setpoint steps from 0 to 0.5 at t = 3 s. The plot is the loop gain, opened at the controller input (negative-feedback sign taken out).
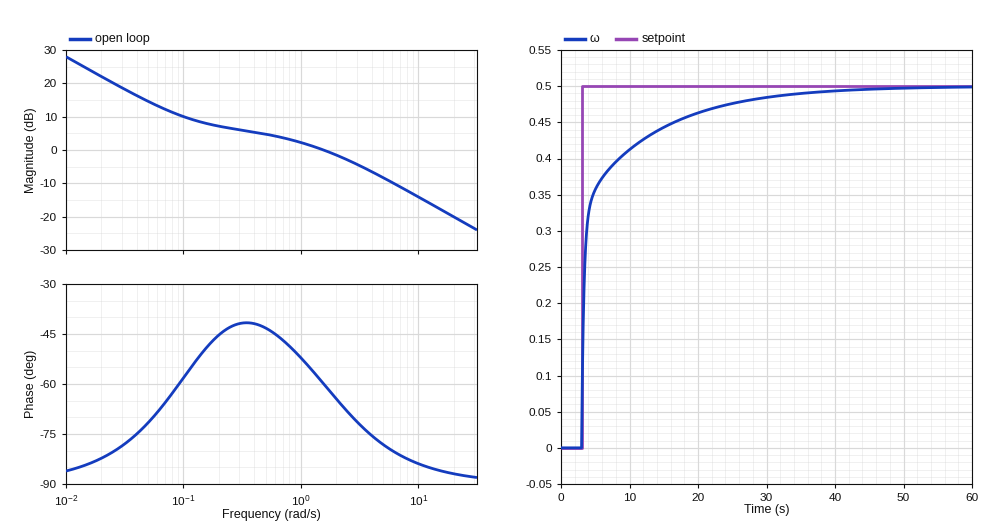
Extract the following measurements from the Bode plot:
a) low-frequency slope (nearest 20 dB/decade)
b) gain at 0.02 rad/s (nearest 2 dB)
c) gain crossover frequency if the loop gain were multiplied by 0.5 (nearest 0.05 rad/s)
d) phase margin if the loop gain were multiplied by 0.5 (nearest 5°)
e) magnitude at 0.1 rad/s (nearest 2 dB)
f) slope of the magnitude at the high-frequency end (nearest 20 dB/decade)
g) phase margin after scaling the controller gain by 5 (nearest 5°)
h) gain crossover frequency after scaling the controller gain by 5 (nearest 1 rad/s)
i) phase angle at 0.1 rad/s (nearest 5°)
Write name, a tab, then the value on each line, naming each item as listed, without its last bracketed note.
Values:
low-frequency slope	-20 dB/decade
gain at 0.02 rad/s	22 dB
gain crossover frequency if the loop gain were multiplied by 0.5	0.30 rad/s
phase margin if the loop gain were multiplied by 0.5	140°
magnitude at 0.1 rad/s	10 dB
slope of the magnitude at the high-frequency end	-20 dB/decade
phase margin after scaling the controller gain by 5	95°
gain crossover frequency after scaling the controller gain by 5	10 rad/s
phase angle at 0.1 rad/s	-60°
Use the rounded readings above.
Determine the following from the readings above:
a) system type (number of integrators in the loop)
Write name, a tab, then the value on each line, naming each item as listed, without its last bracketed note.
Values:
system type	1
